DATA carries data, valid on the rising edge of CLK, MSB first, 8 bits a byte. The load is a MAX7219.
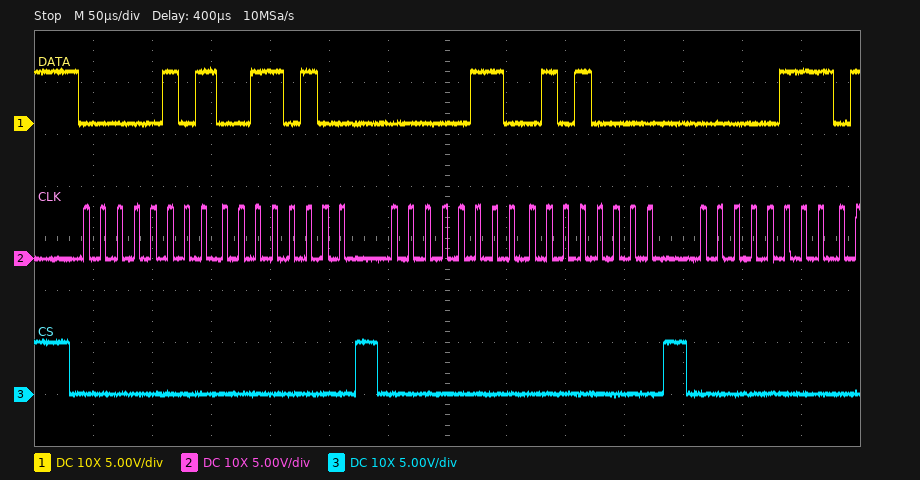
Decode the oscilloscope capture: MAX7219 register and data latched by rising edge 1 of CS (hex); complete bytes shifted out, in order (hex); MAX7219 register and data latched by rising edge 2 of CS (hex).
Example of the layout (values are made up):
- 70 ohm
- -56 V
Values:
- register 0x5, data 0x34
- 05 34 06 50 07
- register 0x6, data 0x50
